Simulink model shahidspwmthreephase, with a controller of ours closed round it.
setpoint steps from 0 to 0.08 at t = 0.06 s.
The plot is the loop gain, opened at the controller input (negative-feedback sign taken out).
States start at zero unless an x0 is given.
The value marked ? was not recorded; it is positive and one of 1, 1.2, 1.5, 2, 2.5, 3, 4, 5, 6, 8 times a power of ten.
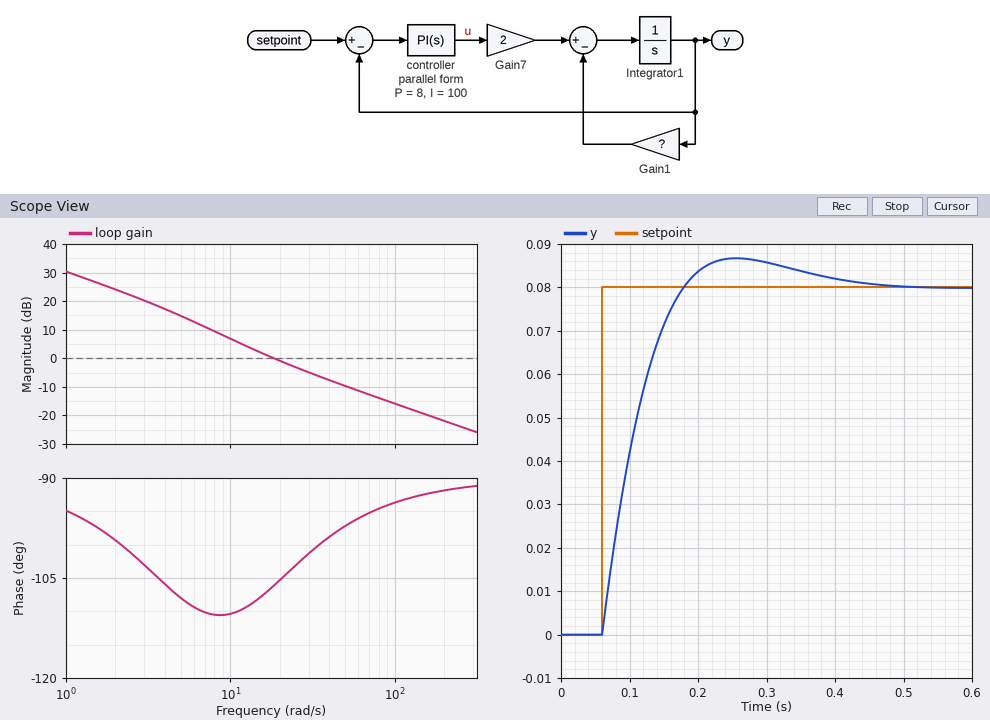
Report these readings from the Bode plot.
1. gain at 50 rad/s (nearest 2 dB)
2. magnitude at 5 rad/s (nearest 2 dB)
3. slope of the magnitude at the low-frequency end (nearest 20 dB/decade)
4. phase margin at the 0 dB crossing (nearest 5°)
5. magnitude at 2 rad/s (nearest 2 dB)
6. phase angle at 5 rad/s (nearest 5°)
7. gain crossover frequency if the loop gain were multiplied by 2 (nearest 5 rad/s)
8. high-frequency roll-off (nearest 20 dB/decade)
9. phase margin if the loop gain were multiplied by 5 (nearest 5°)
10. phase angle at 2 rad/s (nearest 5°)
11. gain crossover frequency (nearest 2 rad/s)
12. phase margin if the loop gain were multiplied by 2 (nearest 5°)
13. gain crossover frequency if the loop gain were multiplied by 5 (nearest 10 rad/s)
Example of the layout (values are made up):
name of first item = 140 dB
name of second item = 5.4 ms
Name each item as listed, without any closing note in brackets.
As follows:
gain at 50 rad/s = -10 dB
magnitude at 5 rad/s = 14 dB
slope of the magnitude at the low-frequency end = -20 dB/decade
phase margin at the 0 dB crossing = 75°
magnitude at 2 rad/s = 24 dB
phase angle at 5 rad/s = -110°
gain crossover frequency if the loop gain were multiplied by 2 = 35 rad/s
high-frequency roll-off = -20 dB/decade
phase margin if the loop gain were multiplied by 5 = 85°
phase angle at 2 rad/s = -100°
gain crossover frequency = 18 rad/s
phase margin if the loop gain were multiplied by 2 = 80°
gain crossover frequency if the loop gain were multiplied by 5 = 80 rad/s
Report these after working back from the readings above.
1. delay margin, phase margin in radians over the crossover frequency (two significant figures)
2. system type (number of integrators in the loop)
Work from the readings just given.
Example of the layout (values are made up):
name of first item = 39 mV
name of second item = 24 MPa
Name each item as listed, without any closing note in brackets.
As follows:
delay margin, phase margin in radians over the crossover frequency = 0.073 s
system type = 1
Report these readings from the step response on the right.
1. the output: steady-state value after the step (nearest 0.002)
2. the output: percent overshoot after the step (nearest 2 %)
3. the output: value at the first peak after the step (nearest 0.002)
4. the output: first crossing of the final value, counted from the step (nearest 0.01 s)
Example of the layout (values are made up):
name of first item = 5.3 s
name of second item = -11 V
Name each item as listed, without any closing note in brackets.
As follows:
the output: steady-state value after the step = 0.080
the output: percent overshoot after the step = 8 %
the output: value at the first peak after the step = 0.086
the output: first crossing of the final value, counted from the step = 0.12 s
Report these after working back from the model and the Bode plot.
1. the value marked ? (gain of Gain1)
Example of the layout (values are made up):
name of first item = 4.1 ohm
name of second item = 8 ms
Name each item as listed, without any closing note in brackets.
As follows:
the value marked ? = 6
